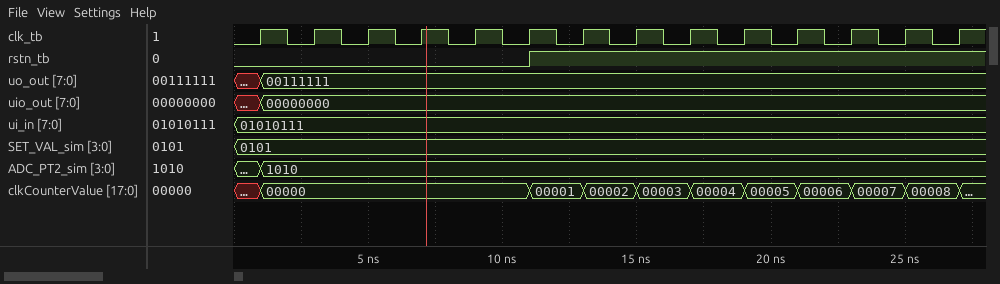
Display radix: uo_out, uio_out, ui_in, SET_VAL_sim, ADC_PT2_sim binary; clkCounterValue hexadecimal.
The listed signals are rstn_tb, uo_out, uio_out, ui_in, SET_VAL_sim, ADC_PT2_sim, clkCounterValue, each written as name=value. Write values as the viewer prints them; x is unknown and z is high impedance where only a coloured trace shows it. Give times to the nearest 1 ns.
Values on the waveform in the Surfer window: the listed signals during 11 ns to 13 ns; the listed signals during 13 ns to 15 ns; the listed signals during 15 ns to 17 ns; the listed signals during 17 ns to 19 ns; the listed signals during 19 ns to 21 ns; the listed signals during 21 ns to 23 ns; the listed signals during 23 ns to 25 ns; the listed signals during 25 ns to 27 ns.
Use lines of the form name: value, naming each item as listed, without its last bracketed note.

the listed signals during 11 ns to 13 ns: rstn_tb=1, uo_out=00111111, uio_out=00000000, ui_in=01010111, SET_VAL_sim=0101, ADC_PT2_sim=1010, clkCounterValue=00001
the listed signals during 13 ns to 15 ns: rstn_tb=1, uo_out=00111111, uio_out=00000000, ui_in=01010111, SET_VAL_sim=0101, ADC_PT2_sim=1010, clkCounterValue=00002
the listed signals during 15 ns to 17 ns: rstn_tb=1, uo_out=00111111, uio_out=00000000, ui_in=01010111, SET_VAL_sim=0101, ADC_PT2_sim=1010, clkCounterValue=00003
the listed signals during 17 ns to 19 ns: rstn_tb=1, uo_out=00111111, uio_out=00000000, ui_in=01010111, SET_VAL_sim=0101, ADC_PT2_sim=1010, clkCounterValue=00004
the listed signals during 19 ns to 21 ns: rstn_tb=1, uo_out=00111111, uio_out=00000000, ui_in=01010111, SET_VAL_sim=0101, ADC_PT2_sim=1010, clkCounterValue=00005
the listed signals during 21 ns to 23 ns: rstn_tb=1, uo_out=00111111, uio_out=00000000, ui_in=01010111, SET_VAL_sim=0101, ADC_PT2_sim=1010, clkCounterValue=00006
the listed signals during 23 ns to 25 ns: rstn_tb=1, uo_out=00111111, uio_out=00000000, ui_in=01010111, SET_VAL_sim=0101, ADC_PT2_sim=1010, clkCounterValue=00007
the listed signals during 25 ns to 27 ns: rstn_tb=1, uo_out=00111111, uio_out=00000000, ui_in=01010111, SET_VAL_sim=0101, ADC_PT2_sim=1010, clkCounterValue=00008
